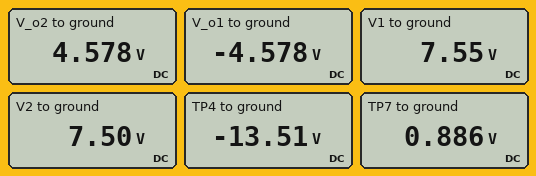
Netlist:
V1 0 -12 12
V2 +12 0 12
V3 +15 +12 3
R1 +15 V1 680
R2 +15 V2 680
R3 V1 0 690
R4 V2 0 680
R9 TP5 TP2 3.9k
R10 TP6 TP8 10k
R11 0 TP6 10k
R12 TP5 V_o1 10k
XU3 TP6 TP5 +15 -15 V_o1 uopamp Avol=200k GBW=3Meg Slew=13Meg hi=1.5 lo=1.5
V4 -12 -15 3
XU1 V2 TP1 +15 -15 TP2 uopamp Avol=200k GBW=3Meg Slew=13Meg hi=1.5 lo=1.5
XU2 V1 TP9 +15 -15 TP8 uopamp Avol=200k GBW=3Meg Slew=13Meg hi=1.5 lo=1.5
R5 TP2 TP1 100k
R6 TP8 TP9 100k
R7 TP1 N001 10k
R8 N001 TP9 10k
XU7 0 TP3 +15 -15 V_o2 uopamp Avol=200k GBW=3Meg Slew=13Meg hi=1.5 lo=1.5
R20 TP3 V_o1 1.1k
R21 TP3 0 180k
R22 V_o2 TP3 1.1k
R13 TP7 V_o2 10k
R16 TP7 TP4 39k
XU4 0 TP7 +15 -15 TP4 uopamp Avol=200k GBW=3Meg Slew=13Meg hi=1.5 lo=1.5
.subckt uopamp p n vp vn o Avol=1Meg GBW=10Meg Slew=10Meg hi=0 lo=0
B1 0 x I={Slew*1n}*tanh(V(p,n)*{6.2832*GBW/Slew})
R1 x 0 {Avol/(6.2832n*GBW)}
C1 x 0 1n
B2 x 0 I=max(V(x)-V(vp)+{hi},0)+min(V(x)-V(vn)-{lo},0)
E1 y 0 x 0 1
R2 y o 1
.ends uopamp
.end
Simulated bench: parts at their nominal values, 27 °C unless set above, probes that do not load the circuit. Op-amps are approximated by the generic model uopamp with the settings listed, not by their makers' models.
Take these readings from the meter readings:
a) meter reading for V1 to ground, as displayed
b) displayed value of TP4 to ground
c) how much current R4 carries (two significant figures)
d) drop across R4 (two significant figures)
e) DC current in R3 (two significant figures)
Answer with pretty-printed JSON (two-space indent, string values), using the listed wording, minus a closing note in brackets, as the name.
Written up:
{
  "meter reading for V1 to ground, as displayed": "7.55 V",
  "displayed value of TP4 to ground": "-13.51 V",
  "how much current R4 carries": "11 mA",
  "drop across R4": "7.5 V",
  "DC current in R3": "11 mA"
}
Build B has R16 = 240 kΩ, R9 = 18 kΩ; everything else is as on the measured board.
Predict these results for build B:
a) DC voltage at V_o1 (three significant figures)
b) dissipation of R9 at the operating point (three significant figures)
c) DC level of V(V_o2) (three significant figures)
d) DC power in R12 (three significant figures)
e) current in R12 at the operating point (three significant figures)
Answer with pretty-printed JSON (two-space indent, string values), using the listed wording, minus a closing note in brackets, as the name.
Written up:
{
  "DC voltage at V_o1": "2.07 V",
  "dissipation of R9 at the operating point": "609 µW",
  "DC level of V(V_o2)": "-2.07 V",
  "DC power in R12": "339 µW",
  "current in R12 at the operating point": "184 µA"
}
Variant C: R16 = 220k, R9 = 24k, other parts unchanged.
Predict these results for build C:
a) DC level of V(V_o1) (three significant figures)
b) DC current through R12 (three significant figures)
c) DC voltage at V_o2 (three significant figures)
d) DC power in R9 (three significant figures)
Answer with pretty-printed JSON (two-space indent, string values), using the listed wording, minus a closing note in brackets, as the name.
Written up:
{
  "DC level of V(V_o1)": "2.53 V",
  "DC current through R12": "138 µA",
  "DC voltage at V_o2": "-2.53 V",
  "DC power in R9": "457 µW"
}
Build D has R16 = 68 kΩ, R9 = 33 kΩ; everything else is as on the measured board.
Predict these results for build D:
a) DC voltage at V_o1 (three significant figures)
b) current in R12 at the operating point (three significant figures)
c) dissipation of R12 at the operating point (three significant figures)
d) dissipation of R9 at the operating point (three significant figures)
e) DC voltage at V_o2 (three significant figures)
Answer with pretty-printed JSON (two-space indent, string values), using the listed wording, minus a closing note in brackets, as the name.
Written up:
{
  "DC voltage at V_o1": "2.91 V",
  "current in R12 at the operating point": "100 µA",
  "dissipation of R12 at the operating point": "101 µW",
  "dissipation of R9 at the operating point": "332 µW",
  "DC voltage at V_o2": "-2.91 V"
}
